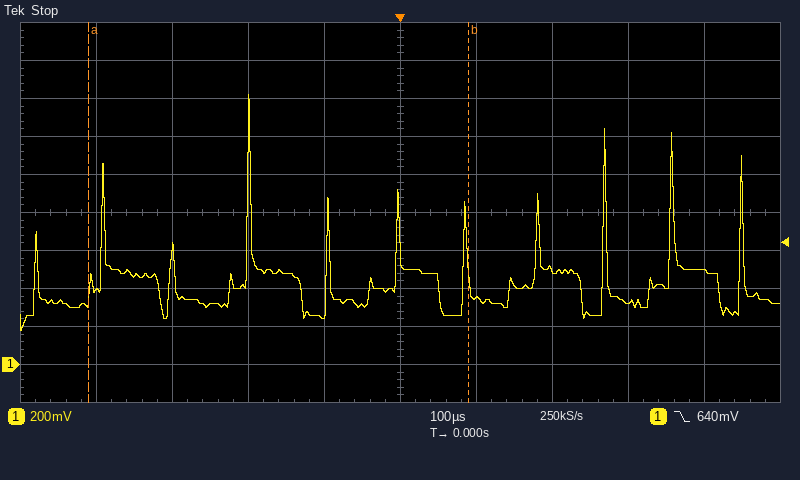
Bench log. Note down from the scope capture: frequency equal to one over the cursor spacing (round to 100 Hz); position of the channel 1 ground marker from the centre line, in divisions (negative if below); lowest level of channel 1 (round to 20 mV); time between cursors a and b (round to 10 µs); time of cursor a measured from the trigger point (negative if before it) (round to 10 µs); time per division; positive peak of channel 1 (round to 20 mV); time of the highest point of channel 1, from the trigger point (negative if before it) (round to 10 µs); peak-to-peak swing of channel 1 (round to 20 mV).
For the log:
2.0 kHz
-4.0 div
180 mV
500 µs
-410 µs
100 µs
1.42 V
-200 µs
1.24 V
